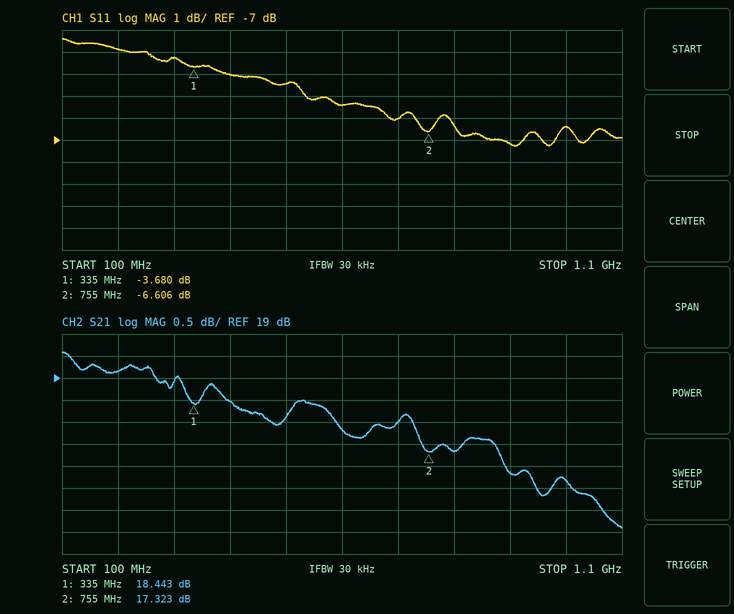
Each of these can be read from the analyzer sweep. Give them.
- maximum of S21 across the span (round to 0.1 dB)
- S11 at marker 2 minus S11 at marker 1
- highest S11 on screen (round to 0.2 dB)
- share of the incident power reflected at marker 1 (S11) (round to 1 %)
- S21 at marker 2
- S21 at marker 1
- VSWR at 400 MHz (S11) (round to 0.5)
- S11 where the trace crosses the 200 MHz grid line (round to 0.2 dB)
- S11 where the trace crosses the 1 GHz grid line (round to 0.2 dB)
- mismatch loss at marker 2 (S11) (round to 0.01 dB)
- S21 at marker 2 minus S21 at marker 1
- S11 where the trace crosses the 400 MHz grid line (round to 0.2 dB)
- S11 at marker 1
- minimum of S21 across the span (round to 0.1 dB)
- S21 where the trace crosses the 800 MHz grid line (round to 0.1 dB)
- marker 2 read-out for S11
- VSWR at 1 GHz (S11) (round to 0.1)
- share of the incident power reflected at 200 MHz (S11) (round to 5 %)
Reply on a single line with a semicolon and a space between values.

19.6 dB; -2.926 dB; -2.4 dB; 43 %; 17.323 dB; 18.443 dB; 4.5; -2.8 dB; -6.4 dB; 1.07 dB; -1.120 dB; -4.0 dB; -3.680 dB; 15.6 dB; 17.3 dB; -6.606 dB; 2.8; 50 %
